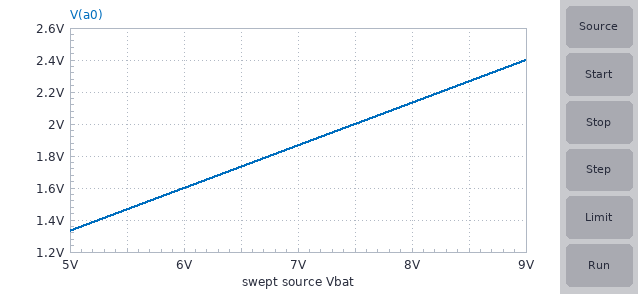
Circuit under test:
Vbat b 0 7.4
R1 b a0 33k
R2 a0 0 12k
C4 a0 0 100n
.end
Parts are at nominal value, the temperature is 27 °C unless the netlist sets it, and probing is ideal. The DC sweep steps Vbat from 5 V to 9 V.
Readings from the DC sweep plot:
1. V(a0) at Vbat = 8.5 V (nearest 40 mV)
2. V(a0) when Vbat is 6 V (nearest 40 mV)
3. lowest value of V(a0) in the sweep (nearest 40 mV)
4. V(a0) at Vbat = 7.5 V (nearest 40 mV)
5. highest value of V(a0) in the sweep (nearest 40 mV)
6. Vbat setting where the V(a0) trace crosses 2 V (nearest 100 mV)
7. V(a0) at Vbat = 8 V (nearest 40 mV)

2.28 V
1.60 V
1.32 V
2.00 V
2.40 V
7.5 V
2.12 V
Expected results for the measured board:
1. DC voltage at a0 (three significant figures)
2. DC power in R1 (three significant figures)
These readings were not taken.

1.97 V
892 µW
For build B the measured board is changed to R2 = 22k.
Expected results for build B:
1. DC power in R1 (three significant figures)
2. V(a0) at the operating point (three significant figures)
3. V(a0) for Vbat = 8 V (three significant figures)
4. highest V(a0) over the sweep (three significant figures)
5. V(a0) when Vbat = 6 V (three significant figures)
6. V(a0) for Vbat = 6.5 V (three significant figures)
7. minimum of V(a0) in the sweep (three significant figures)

597 µW
2.96 V
3.20 V
3.60 V
2.40 V
2.60 V
2.00 V
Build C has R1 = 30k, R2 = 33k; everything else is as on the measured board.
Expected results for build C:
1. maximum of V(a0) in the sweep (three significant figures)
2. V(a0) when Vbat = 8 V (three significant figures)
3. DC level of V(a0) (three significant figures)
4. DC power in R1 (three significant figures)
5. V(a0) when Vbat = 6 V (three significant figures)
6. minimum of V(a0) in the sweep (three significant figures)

4.71 V
4.19 V
3.88 V
414 µW
3.14 V
2.62 V
